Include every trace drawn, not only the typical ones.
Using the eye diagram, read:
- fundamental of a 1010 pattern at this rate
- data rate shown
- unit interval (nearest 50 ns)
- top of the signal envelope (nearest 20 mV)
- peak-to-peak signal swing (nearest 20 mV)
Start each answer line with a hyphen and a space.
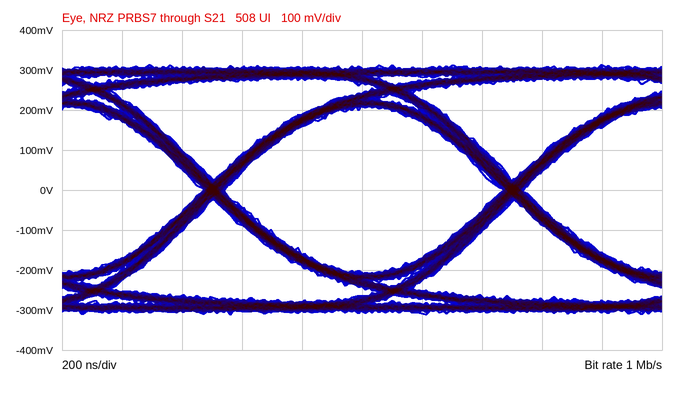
- 500 kHz
- 1 Mb/s
- 1.00 µs
- 320 mV
- 620 mV
